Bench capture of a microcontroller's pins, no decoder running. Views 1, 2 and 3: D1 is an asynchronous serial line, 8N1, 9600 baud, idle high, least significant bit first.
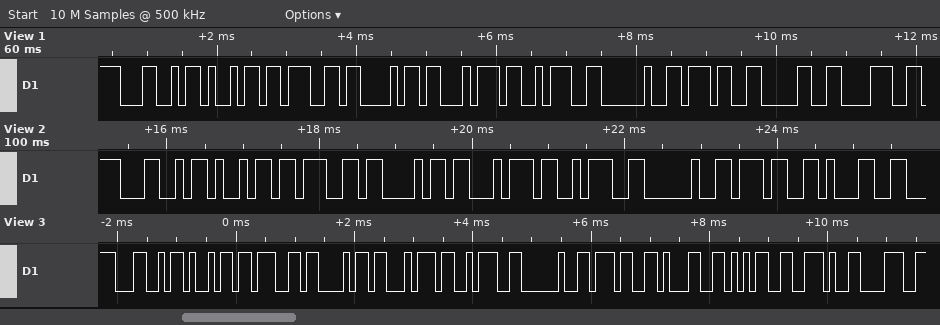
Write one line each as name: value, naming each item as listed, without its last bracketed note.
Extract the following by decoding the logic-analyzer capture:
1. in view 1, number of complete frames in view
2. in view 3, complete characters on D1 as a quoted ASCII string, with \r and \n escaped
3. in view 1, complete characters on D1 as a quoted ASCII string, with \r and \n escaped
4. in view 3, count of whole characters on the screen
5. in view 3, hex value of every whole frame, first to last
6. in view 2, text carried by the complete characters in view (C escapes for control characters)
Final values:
in view 1, number of complete frames in view: 10
in view 3, complete characters on D1 as a quoted ASCII string, with \r and \n escaped: "Light: 715.8"
in view 1, complete characters on D1 as a quoted ASCII string, with \r and \n escaped: "Light: 708"
in view 3, count of whole characters on the screen: 12
in view 3, hex value of every whole frame, first to last: 4C 69 67 68 74 3A 20 37 31 35 2E 38
in view 2, text carried by the complete characters in view: "Light: 71"
